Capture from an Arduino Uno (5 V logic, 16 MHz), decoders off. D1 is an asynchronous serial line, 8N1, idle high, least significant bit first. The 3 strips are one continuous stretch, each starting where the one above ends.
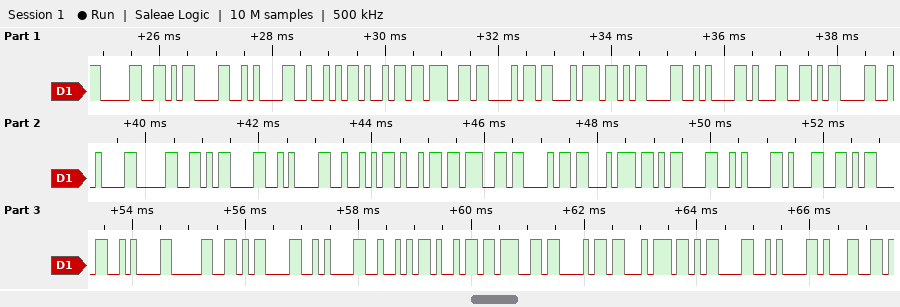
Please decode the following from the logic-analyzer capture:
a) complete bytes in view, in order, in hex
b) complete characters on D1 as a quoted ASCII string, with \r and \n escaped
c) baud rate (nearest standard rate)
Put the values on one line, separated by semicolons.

30 0D 0A 52 69 67 68 74 0D 0A 31 0D 0A 30 0D 0A 52 69 67 68 74 0D 0A 31 0D 0A 30 0D 0A 52 69 67 68 74 0D 0A 31; "0\r\nRight\r\n1\r\n0\r\nRight\r\n1\r\n0\r\nRight\r\n1"; 9600 baud
